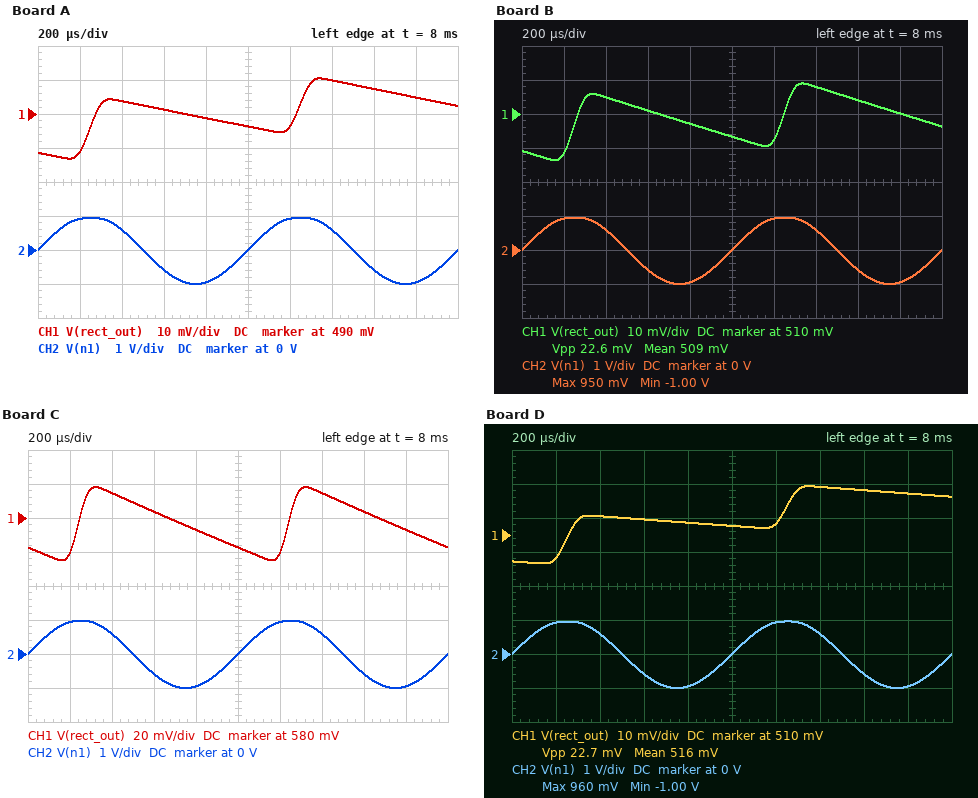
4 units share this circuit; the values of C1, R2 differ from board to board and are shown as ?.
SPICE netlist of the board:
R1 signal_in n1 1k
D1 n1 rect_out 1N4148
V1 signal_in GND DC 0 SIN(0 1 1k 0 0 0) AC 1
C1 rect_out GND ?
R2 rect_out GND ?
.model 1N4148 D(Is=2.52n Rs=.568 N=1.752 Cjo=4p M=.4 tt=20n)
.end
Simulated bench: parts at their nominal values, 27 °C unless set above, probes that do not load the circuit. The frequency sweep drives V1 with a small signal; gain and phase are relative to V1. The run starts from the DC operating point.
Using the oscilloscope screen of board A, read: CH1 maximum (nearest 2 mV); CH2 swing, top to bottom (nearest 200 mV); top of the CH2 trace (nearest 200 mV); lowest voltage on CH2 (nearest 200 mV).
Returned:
500 mV
2.0 V
1.0 V
-1.0 V
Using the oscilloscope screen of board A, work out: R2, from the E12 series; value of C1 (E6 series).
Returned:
120 kΩ
330 nF
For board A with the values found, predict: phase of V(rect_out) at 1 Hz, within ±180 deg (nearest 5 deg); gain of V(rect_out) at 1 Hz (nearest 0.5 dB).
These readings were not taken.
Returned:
-15 deg
-44.0 dB
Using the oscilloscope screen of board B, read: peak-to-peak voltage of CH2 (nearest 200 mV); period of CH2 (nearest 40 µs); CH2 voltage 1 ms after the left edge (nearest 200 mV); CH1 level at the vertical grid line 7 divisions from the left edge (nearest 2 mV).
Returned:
2.0 V
1.00 ms
0 V
518 mV
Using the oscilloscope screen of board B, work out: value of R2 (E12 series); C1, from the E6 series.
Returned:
120 kΩ
220 nF
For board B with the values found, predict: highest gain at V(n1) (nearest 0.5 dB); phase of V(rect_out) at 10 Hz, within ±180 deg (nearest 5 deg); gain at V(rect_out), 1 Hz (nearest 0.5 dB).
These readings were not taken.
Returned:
0 dB
-60 deg
-43.5 dB
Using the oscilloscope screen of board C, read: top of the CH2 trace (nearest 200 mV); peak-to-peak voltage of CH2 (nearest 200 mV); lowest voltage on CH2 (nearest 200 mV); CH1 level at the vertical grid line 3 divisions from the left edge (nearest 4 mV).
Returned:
1.0 V
2.0 V
-1.0 V
584 mV
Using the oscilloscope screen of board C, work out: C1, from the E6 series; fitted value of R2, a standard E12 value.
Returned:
33 nF
330 kΩ
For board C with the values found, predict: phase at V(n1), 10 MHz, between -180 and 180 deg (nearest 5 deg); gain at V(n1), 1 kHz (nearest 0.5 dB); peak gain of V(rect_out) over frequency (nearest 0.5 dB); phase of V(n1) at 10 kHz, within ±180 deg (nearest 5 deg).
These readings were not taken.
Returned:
-15 deg
0 dB
-35.0 dB
0 deg
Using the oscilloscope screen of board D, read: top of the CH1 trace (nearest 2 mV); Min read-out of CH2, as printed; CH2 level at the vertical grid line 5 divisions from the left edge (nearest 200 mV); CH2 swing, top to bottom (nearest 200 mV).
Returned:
524 mV
-1.00 V
0 V
2.0 V
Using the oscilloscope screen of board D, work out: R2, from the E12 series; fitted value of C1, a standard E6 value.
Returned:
330 kΩ
330 nF
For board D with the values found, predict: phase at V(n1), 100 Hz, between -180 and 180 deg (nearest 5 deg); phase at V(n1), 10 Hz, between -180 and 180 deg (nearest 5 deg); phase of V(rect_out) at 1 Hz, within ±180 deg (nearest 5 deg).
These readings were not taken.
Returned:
0 deg
0 deg
-35 deg
